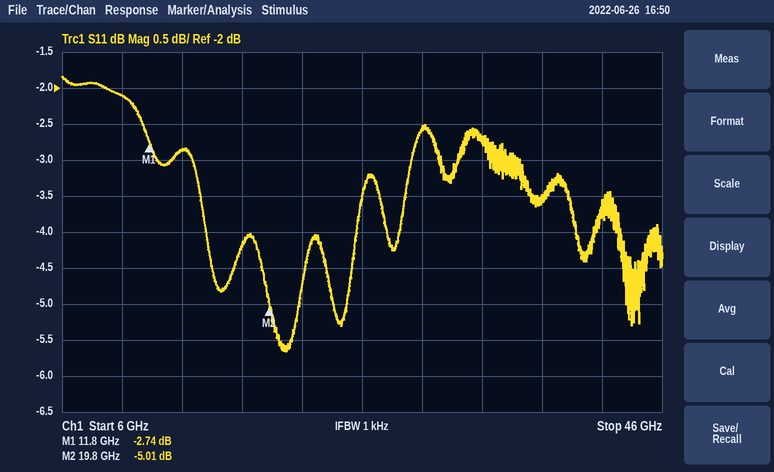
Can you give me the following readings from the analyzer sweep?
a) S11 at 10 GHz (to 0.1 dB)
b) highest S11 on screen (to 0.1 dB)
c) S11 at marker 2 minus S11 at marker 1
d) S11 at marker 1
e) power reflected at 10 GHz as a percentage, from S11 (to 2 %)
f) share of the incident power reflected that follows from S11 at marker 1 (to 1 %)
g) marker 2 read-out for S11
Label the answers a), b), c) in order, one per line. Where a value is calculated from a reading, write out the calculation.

a) -2.1 dB
b) -1.8 dB
c) -5.01 − (-2.74) = -2.27 dB
d) -2.74 dB
e) 10^(-2.1/10) ≈ 62 %
f) 10^(-2.74/10) ≈ 53 %
g) -5.01 dB
